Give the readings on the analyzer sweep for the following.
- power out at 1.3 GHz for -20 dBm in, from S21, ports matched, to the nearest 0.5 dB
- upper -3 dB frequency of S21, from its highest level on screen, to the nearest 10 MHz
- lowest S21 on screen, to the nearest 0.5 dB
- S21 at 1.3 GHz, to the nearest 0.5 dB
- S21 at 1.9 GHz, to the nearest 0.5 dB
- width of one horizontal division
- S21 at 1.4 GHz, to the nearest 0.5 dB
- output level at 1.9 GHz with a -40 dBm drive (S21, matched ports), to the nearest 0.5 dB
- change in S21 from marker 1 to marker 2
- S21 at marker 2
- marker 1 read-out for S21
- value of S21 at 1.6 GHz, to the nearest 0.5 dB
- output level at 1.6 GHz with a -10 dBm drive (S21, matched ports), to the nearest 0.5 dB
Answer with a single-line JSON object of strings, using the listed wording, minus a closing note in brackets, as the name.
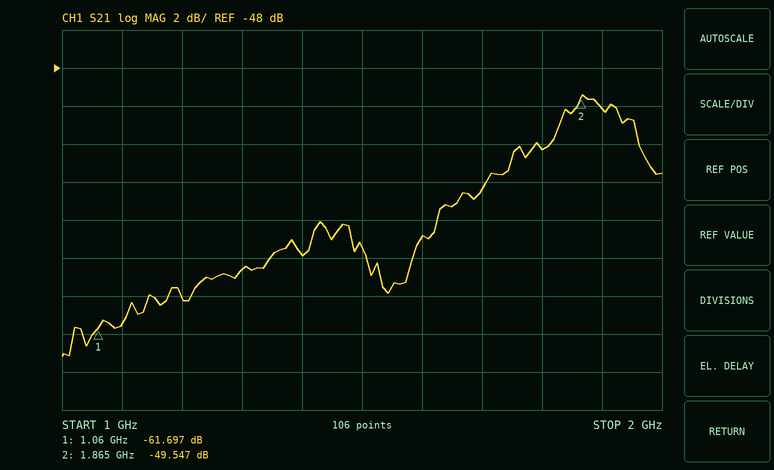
{"power out at 1.3 GHz for -20 dBm in, from S21, ports matched, to the nearest 0.5 dB": "-78.5 dBm", "upper -3 dB frequency of S21, from its highest level on screen, to the nearest 10 MHz": "1.97 GHz", "lowest S21 on screen, to the nearest 0.5 dB": "-63.0 dB", "S21 at 1.3 GHz, to the nearest 0.5 dB": "-58.5 dB", "S21 at 1.9 GHz, to the nearest 0.5 dB": "-50.0 dB", "width of one horizontal division": "100 MHz", "S21 at 1.4 GHz, to the nearest 0.5 dB": "-58.0 dB", "output level at 1.9 GHz with a -40 dBm drive (S21, matched ports), to the nearest 0.5 dB": "-90.0 dBm", "change in S21 from marker 1 to marker 2": "12.150 dB", "S21 at marker 2": "-49.547 dB", "marker 1 read-out for S21": "-61.697 dB", "value of S21 at 1.6 GHz, to the nearest 0.5 dB": "-57.0 dB", "output level at 1.6 GHz with a -10 dBm drive (S21, matched ports), to the nearest 0.5 dB": "-67.0 dBm"}
